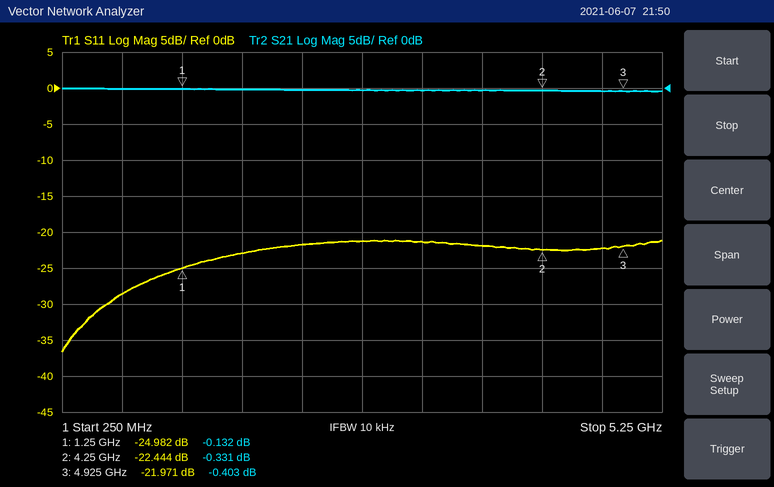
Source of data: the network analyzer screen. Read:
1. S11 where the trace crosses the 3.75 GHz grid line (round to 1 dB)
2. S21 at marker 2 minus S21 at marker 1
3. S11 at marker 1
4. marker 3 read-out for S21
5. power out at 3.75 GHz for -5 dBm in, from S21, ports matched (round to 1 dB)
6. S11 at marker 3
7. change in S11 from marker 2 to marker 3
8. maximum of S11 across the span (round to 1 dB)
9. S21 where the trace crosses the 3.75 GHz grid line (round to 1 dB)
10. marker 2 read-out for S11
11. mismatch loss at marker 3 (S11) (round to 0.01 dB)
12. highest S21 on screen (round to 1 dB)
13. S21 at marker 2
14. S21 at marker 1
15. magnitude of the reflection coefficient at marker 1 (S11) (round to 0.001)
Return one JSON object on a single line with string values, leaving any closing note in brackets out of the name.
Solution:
{"S11 where the trace crosses the 3.75 GHz grid line": "-22 dB", "S21 at marker 2 minus S21 at marker 1": "-0.199 dB", "S11 at marker 1": "-24.982 dB", "marker 3 read-out for S21": "-0.403 dB", "power out at 3.75 GHz for -5 dBm in, from S21, ports matched": "-5 dBm", "S11 at marker 3": "-21.971 dB", "change in S11 from marker 2 to marker 3": "0.473 dB", "maximum of S11 across the span": "-21 dB", "S21 where the trace crosses the 3.75 GHz grid line": "0 dB", "marker 2 read-out for S11": "-22.444 dB", "mismatch loss at marker 3 (S11)": "0.03 dB", "highest S21 on screen": "0 dB", "S21 at marker 2": "-0.331 dB", "S21 at marker 1": "-0.132 dB", "magnitude of the reflection coefficient at marker 1 (S11)": "0.056"}
